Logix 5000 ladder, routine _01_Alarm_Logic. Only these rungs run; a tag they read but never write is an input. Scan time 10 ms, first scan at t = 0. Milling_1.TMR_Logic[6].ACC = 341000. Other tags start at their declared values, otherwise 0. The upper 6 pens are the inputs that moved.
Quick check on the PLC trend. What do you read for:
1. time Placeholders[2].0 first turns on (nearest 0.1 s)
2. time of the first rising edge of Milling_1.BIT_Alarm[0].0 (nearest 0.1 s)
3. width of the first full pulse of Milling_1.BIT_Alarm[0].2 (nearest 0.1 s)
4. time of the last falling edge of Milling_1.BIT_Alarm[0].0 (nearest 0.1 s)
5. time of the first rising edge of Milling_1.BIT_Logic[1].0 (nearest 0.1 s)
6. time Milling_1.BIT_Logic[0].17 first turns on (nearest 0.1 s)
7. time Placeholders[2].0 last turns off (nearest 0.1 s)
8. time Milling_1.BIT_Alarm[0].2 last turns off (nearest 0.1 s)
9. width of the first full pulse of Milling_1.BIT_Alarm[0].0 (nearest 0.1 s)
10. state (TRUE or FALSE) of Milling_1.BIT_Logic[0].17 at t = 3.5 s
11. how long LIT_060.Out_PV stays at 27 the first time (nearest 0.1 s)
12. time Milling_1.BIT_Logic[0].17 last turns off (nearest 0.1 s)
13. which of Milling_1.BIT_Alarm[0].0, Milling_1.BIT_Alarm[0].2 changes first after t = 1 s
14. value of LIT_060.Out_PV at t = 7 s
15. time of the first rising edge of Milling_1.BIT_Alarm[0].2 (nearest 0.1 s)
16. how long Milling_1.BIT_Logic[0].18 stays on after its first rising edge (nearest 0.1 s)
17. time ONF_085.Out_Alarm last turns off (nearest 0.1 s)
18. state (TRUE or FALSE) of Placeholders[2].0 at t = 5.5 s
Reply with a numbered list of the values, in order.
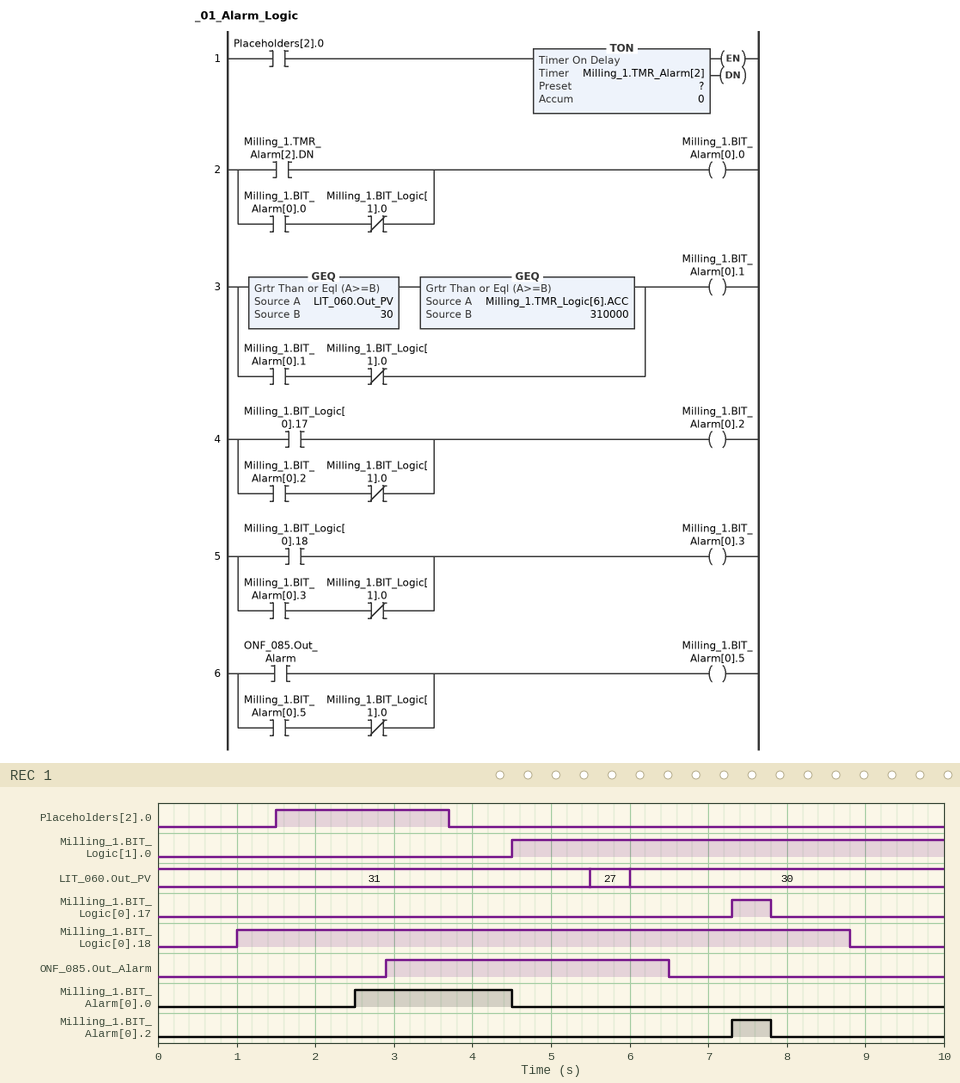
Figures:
1. 1.5 s
2. 2.5 s
3. 0.5 s
4. 4.5 s
5. 4.5 s
6. 7.3 s
7. 3.7 s
8. 7.8 s
9. 2.0 s
10. FALSE
11. 0.5 s
12. 7.8 s
13. Milling_1.BIT_Alarm[0].0
14. 30
15. 7.3 s
16. 7.8 s
17. 6.5 s
18. FALSE
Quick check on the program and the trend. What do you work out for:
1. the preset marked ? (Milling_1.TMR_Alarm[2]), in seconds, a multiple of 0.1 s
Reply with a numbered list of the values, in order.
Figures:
1. 1.0 s
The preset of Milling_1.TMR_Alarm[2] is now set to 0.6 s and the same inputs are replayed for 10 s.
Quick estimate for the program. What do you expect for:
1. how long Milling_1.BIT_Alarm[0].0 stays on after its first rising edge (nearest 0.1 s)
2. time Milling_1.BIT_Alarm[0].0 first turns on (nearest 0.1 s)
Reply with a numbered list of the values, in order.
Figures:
1. 2.4 s
2. 2.1 s
